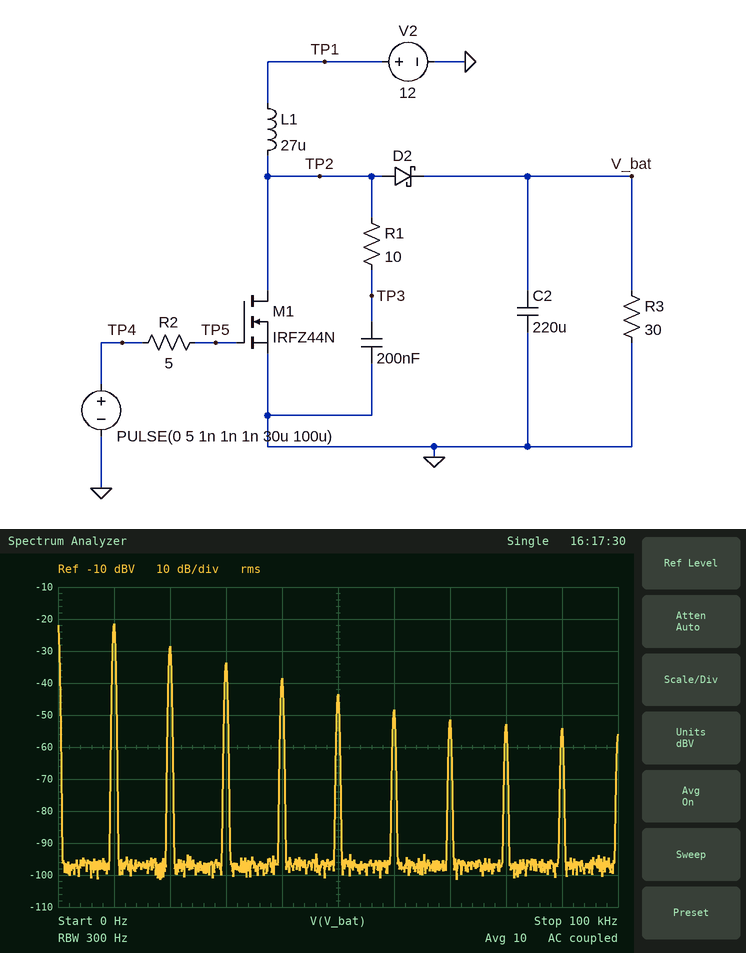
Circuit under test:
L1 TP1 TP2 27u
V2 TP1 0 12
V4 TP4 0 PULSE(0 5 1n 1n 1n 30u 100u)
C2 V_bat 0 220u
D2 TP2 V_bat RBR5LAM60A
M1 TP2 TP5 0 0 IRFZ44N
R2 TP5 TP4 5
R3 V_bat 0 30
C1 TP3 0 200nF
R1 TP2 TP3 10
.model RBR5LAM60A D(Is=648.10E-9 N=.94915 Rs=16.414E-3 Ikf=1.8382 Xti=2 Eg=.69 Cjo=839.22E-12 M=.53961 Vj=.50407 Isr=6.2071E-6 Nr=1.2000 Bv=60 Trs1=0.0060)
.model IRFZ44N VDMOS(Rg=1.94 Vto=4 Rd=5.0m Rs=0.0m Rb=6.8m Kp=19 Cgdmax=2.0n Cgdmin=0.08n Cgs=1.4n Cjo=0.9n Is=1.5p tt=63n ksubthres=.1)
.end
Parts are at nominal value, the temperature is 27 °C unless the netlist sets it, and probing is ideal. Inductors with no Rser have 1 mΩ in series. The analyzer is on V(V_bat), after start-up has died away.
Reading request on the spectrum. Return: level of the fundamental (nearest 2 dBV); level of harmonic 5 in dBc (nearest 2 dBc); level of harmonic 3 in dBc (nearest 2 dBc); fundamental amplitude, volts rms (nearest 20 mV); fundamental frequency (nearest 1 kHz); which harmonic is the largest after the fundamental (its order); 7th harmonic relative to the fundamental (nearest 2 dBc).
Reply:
-22 dBV
-22 dBc
-12 dBc
80 mV
10 kHz
2
-30 dBc
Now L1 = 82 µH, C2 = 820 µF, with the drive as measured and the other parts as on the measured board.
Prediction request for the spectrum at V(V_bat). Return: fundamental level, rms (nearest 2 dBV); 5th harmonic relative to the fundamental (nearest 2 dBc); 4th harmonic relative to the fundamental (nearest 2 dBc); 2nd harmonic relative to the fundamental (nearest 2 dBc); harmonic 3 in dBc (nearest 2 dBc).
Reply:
-36 dBV
-28 dBc
-24 dBc
-10 dBc
-20 dBc
